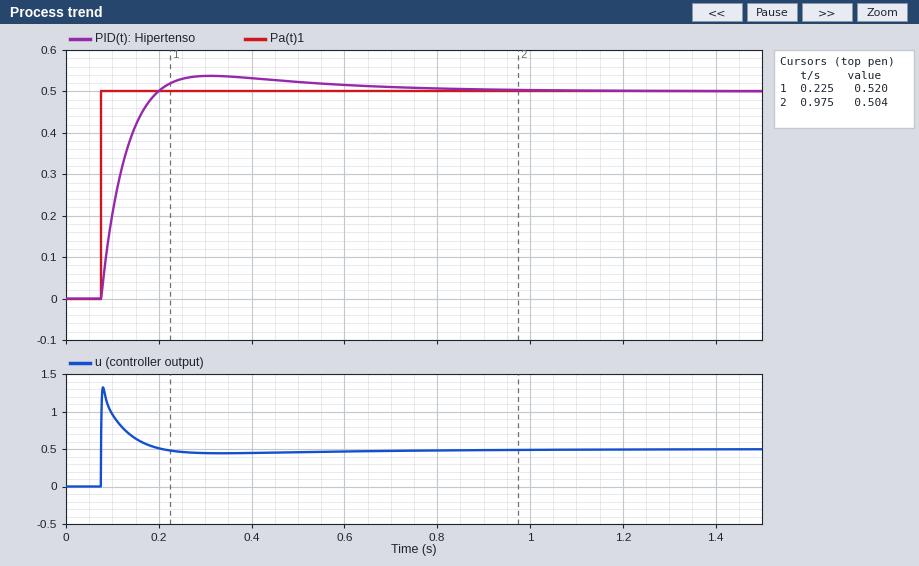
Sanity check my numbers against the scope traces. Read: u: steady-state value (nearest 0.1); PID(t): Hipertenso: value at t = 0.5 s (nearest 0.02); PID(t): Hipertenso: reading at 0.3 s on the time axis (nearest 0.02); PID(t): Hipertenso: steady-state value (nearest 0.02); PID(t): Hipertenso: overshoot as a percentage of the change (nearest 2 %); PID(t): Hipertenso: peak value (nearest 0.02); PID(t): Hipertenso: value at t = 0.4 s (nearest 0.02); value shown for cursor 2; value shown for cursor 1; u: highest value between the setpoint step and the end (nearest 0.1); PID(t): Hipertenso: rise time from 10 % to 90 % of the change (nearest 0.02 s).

0.5
0.52
0.54
0.50
8 %
0.54
0.54
0.504
0.520
1.3
0.08 s
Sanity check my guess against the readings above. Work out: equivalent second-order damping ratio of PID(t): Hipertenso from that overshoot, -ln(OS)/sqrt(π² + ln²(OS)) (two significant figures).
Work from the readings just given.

0.63
